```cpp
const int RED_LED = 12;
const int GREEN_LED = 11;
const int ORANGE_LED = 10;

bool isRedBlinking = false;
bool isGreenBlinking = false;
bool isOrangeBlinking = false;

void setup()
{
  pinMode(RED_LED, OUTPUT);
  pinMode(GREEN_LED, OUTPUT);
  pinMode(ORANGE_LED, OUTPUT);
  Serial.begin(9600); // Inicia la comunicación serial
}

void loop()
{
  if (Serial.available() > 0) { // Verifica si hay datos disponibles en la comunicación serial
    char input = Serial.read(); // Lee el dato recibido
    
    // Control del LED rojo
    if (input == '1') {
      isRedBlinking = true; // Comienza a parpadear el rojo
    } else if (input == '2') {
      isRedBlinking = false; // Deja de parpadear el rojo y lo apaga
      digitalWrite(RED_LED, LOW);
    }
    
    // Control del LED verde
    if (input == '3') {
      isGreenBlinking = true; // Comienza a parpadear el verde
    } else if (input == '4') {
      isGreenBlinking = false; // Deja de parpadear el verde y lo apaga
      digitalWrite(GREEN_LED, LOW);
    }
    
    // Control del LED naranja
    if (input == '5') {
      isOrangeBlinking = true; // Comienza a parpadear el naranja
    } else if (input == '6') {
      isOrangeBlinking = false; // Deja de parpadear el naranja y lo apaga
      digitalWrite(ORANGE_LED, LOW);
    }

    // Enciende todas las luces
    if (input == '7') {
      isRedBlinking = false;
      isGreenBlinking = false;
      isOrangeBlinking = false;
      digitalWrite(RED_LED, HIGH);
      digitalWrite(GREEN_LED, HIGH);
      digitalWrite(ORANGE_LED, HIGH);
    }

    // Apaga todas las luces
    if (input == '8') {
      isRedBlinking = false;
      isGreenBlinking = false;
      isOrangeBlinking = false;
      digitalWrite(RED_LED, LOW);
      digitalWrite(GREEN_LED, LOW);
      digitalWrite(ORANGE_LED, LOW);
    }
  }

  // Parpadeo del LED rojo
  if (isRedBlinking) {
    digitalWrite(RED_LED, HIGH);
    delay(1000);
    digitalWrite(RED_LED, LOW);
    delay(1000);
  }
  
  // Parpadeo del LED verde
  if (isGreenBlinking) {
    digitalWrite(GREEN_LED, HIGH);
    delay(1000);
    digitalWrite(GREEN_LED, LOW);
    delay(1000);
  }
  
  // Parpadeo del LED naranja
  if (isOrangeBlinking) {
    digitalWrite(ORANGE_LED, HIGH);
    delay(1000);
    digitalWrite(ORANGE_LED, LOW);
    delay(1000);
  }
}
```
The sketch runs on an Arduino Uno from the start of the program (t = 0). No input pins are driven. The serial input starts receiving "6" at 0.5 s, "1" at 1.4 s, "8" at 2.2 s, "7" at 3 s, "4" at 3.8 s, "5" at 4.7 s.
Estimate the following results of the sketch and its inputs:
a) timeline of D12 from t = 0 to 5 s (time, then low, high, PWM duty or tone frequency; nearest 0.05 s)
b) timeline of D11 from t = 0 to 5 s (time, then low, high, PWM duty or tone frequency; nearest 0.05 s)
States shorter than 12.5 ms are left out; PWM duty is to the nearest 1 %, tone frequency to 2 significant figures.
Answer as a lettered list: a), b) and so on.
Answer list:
a) 0 s low; 1.4 s high; 2.4 s low; 3.4 s high
b) 0 s low; 3.4 s high; 3.8 s low
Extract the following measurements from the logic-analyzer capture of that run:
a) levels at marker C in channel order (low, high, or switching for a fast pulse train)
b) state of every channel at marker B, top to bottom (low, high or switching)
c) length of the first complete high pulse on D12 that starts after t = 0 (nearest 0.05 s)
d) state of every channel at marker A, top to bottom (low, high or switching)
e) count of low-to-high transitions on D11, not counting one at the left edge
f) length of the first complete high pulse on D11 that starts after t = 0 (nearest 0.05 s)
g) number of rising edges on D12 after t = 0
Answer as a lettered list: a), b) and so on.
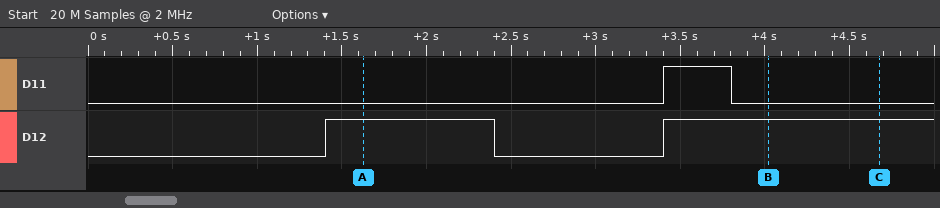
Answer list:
a) D11 low, D12 high
b) D11 low, D12 high
c) 1.00 s
d) D11 low, D12 high
e) 1
f) 0.40 s
g) 2
